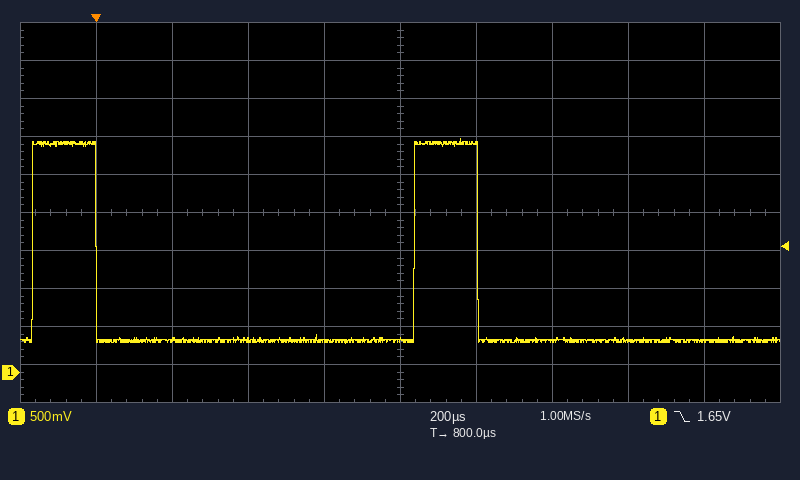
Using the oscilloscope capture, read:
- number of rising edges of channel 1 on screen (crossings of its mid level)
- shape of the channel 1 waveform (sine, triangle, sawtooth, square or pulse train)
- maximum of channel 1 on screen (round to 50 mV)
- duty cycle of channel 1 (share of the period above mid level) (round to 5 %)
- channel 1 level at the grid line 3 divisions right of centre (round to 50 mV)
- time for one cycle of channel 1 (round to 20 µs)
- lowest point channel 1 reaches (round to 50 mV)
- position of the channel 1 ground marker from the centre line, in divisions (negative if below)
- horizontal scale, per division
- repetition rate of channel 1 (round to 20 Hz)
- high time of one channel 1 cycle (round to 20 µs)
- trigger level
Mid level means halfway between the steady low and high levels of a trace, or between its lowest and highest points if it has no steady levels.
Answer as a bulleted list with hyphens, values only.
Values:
- 2
- pulse train
- 3.05 V
- 15 %
- 400 mV
- 1.00 ms
- 400 mV
- -4.2 div
- 200 µs
- 1.00 kHz
- 160 µs
- 1.65 V
